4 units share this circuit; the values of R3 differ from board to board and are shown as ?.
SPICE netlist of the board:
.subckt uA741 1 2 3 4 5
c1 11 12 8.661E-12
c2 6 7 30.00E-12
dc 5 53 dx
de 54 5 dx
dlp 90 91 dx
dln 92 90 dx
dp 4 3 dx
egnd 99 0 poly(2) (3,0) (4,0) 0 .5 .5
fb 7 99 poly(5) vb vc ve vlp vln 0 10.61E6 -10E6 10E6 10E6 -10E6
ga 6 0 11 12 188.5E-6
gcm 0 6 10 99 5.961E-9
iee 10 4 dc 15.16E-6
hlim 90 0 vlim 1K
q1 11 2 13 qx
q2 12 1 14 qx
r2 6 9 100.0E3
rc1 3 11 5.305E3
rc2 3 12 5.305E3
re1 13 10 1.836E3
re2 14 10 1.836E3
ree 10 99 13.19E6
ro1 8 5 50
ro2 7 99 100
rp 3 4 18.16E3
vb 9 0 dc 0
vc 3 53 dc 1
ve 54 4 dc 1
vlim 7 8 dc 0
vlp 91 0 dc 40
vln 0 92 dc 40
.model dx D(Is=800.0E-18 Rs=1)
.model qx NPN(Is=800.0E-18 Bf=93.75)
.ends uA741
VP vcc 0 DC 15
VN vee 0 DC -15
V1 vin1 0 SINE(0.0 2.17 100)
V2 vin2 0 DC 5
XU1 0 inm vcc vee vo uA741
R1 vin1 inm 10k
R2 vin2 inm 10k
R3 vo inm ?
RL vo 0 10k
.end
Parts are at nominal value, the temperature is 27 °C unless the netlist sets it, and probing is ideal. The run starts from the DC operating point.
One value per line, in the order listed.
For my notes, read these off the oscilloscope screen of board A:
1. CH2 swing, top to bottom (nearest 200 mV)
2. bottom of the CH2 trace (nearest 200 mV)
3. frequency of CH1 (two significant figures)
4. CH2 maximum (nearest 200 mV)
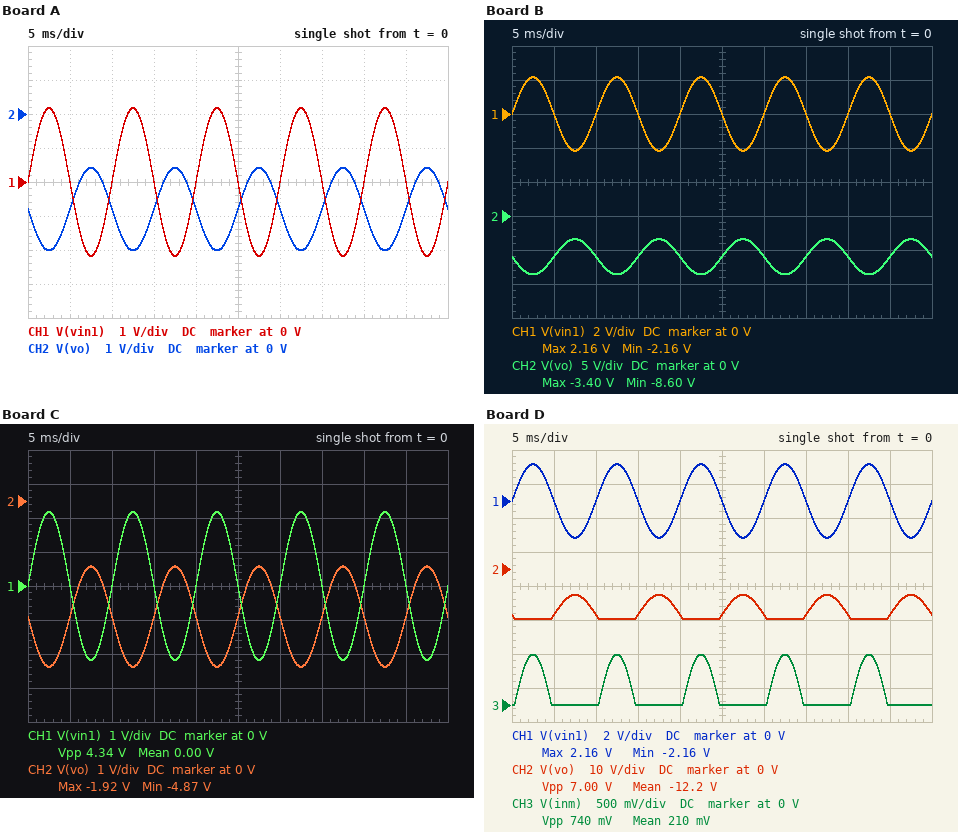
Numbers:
2.4 V
-4.0 V
100 Hz
-1.6 V
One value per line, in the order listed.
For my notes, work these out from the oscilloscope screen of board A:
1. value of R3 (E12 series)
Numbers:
5.6 kΩ
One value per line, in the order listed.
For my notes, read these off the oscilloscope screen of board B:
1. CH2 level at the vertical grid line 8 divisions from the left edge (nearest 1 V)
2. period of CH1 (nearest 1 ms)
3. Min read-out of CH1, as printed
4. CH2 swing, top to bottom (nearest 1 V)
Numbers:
-6 V
10 ms
-2.16 V
5 V
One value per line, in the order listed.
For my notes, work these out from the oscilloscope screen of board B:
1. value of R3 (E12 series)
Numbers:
12 kΩ
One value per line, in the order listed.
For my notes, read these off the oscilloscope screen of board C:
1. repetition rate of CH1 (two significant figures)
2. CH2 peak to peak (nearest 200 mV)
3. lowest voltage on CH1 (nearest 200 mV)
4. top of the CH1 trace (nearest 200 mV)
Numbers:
100 Hz
3.0 V
-2.2 V
2.2 V
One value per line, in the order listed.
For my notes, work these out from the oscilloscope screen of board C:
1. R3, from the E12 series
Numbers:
6.8 kΩ
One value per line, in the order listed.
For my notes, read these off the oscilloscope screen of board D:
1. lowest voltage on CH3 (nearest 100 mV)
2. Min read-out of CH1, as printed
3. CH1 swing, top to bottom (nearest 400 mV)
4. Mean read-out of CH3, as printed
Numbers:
0 V
-2.16 V
4.4 V
210 mV
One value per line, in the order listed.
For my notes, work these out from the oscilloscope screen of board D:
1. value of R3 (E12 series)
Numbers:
27 kΩ
